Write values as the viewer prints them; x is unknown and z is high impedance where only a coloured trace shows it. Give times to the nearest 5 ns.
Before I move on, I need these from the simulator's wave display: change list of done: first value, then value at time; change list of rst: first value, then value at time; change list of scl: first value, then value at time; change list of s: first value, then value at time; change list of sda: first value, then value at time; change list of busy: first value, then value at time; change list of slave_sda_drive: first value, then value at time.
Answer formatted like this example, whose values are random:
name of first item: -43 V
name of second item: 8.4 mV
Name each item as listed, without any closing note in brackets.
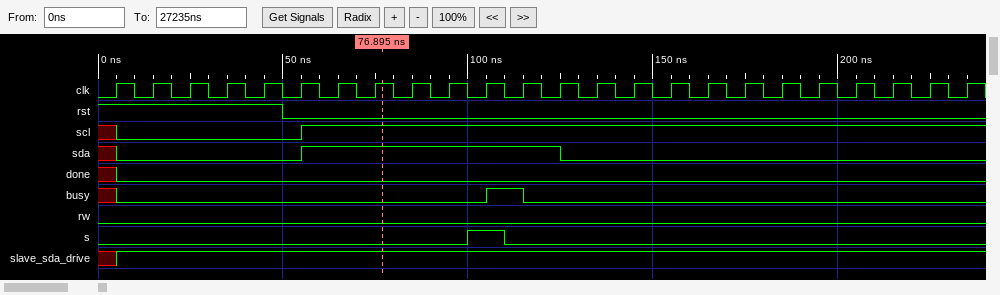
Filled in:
change list of done: first value, then value at time: x, 0 at 5 ns
change list of rst: first value, then value at time: 1, 0 at 50 ns
change list of scl: first value, then value at time: x, 0 at 5 ns, 1 at 55 ns
change list of s: first value, then value at time: 0, 1 at 100 ns, 0 at 110 ns
change list of sda: first value, then value at time: x, 0 at 5 ns, 1 at 55 ns, 0 at 125 ns
change list of busy: first value, then value at time: x, 0 at 5 ns, 1 at 105 ns, 0 at 115 ns
change list of slave_sda_drive: first value, then value at time: x, 1 at 5 ns
